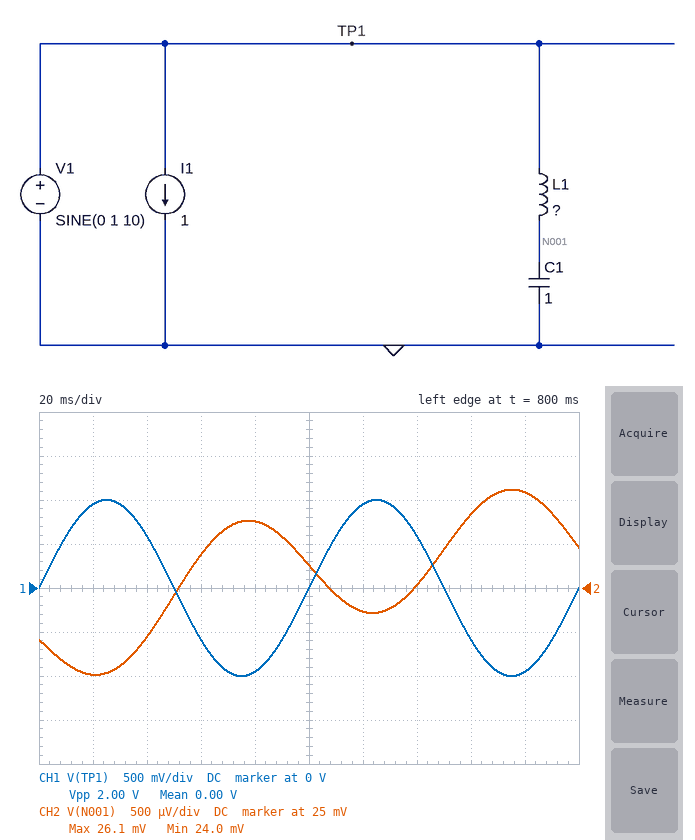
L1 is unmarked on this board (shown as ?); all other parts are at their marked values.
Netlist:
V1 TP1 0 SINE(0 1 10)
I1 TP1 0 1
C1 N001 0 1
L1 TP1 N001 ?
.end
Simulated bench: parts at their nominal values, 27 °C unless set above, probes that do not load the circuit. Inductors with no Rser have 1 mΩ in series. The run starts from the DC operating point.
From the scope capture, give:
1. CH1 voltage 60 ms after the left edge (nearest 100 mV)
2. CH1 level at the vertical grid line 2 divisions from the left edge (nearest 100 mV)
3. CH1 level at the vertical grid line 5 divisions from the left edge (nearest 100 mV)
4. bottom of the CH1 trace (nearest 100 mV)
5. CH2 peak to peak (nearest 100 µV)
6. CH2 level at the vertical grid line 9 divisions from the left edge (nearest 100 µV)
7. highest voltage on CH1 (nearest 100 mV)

-600 mV
600 mV
0 V
-1.0 V
2.1 mV
26.1 mV
1.0 V
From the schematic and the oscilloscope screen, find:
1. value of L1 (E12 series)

390 mH
